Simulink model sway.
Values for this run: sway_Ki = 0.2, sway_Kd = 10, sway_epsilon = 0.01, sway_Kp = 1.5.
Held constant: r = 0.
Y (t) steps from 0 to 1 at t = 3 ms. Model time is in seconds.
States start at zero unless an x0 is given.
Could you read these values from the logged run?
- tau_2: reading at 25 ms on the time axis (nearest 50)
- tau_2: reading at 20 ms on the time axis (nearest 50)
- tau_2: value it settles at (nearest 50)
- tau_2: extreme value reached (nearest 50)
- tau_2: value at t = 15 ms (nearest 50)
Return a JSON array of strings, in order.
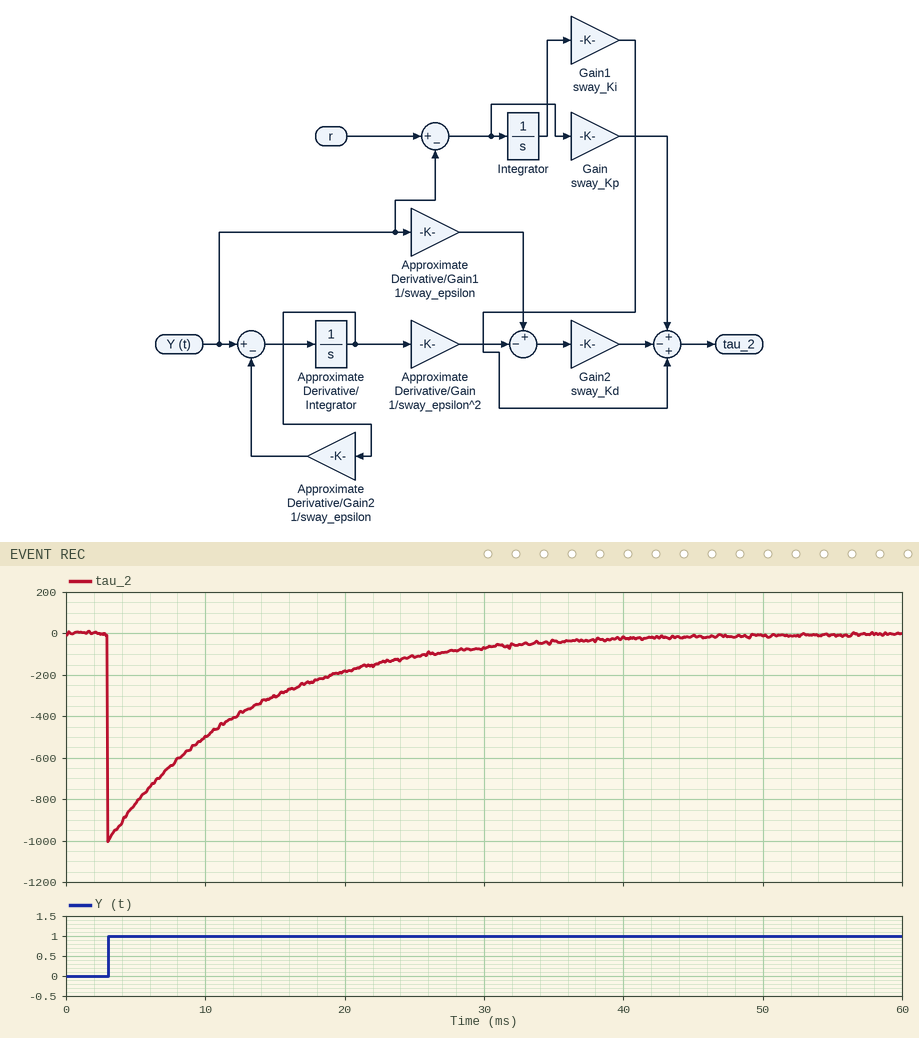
["-100", "-200", "0", "-1000", "-300"]
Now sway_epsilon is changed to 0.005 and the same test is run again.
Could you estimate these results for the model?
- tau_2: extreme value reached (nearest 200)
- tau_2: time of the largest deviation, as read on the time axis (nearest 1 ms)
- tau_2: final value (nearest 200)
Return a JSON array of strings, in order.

["-2000", "3 ms", "0"]
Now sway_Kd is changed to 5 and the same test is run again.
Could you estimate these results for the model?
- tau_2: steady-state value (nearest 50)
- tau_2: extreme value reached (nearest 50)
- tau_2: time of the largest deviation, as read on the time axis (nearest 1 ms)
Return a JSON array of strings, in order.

["0", "-500", "3 ms"]
